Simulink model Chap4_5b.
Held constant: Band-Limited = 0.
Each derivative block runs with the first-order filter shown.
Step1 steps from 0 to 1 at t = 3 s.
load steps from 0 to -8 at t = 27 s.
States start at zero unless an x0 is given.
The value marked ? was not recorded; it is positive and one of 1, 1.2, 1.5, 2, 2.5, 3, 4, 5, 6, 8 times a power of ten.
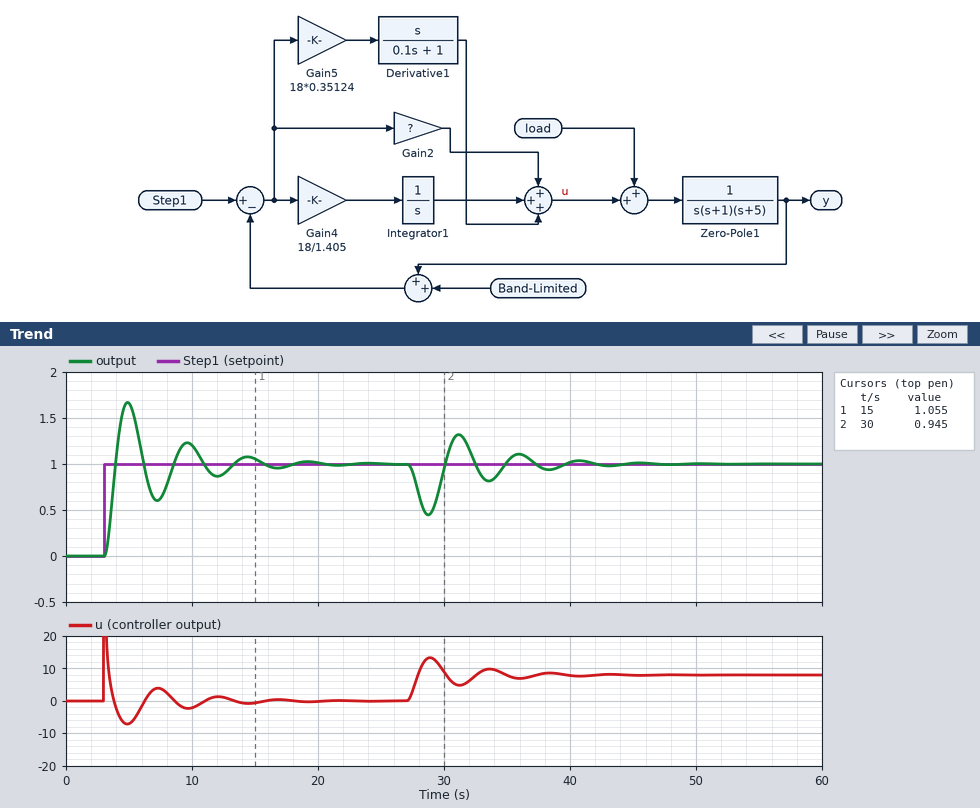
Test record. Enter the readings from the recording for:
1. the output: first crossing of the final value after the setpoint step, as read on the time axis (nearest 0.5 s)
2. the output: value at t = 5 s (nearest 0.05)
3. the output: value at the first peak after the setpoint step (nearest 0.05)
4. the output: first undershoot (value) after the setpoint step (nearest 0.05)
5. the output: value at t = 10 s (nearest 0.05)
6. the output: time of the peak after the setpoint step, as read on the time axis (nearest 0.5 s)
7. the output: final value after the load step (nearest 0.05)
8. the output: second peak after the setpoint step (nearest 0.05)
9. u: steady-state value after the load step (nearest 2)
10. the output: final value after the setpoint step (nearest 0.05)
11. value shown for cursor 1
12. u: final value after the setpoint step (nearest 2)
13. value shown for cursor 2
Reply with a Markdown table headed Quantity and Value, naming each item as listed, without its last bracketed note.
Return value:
| Quantity | Value |
|---|---|
| the output: first crossing of the final value after the setpoint step, as read on the time axis | 4.0 s |
| the output: value at t = 5 s | 1.65 |
| the output: value at the first peak after the setpoint step | 1.65 |
| the output: first undershoot (value) after the setpoint step | 0.60 |
| the output: value at t = 10 s | 1.20 |
| the output: time of the peak after the setpoint step, as read on the time axis | 5.0 s |
| the output: final value after the load step | 1.00 |
| the output: second peak after the setpoint step | 1.25 |
| u: steady-state value after the load step | 8 |
| the output: final value after the setpoint step | 1.00 |
| value shown for cursor 1 | 1.055 |
| u: final value after the setpoint step | 0 |
| value shown for cursor 2 | 0.945 |
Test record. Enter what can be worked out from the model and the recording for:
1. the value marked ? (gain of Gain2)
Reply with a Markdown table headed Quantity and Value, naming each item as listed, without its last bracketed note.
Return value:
| Quantity | Value |
|---|---|
| the value marked ? | 12 |
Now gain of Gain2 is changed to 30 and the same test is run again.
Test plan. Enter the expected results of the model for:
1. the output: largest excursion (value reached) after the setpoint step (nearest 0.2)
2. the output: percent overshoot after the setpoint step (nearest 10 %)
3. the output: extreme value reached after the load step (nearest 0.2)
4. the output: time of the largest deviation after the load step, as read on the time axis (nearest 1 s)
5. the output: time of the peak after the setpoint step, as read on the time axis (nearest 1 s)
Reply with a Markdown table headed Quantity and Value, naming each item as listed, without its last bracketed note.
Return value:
| Quantity | Value |
|---|---|
| the output: largest excursion (value reached) after the setpoint step | 1.8 |
| the output: percent overshoot after the setpoint step | 80 % |
| the output: extreme value reached after the load step | 0.6 |
| the output: time of the largest deviation after the load step, as read on the time axis | 28 s |
| the output: time of the peak after the setpoint step, as read on the time axis | 4 s |
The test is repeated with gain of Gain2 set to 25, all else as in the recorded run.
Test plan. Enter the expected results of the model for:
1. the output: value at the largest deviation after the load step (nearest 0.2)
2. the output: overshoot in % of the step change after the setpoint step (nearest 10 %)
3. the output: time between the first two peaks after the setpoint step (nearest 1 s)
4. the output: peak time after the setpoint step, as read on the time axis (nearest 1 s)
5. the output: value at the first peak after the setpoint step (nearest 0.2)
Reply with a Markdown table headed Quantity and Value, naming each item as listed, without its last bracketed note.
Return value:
| Quantity | Value |
|---|---|
| the output: value at the largest deviation after the load step | 0.6 |
| the output: overshoot in % of the step change after the setpoint step | 80 % |
| the output: time between the first two peaks after the setpoint step | 3 s |
| the output: peak time after the setpoint step, as read on the time axis | 4 s |
| the output: value at the first peak after the setpoint step | 1.8 |
